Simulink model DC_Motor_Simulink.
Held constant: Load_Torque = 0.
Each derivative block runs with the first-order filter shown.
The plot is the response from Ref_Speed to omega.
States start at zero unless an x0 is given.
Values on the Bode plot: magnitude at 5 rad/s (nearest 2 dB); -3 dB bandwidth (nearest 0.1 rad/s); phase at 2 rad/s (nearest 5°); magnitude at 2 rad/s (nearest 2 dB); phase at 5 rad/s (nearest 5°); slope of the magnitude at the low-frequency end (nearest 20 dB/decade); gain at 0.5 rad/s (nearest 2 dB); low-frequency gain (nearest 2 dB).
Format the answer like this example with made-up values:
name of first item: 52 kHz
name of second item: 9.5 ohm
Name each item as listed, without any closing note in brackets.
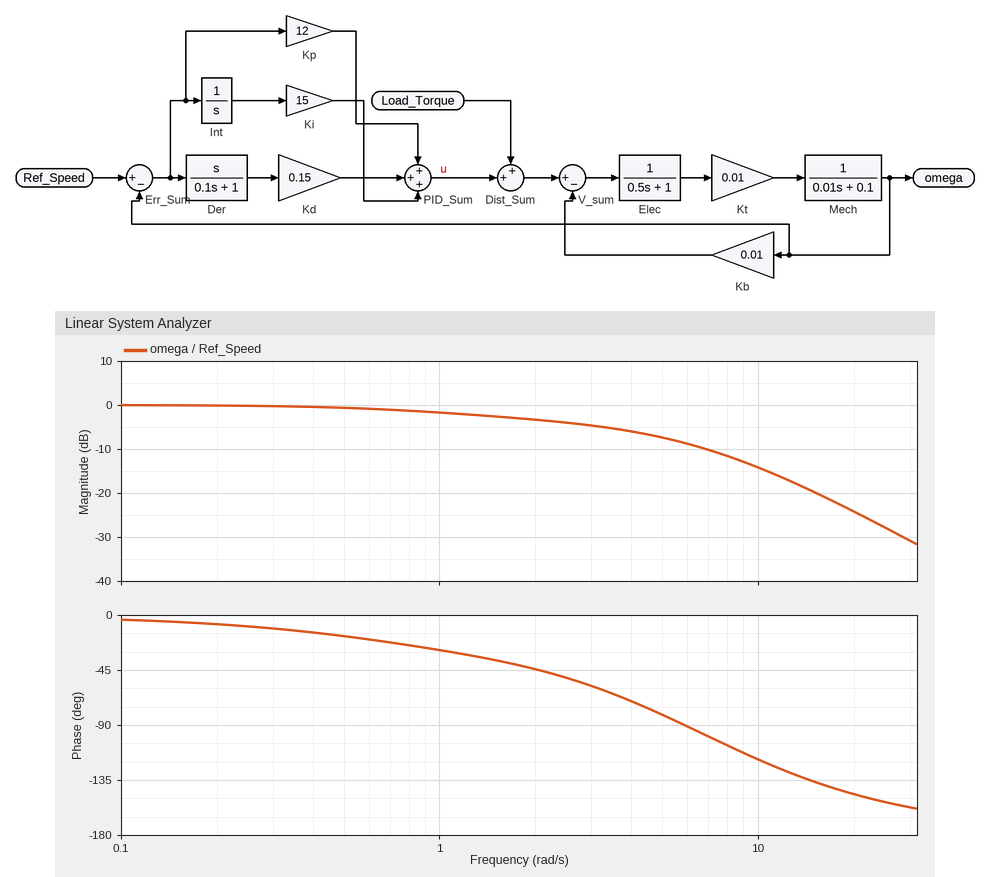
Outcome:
magnitude at 5 rad/s: -8 dB
-3 dB bandwidth: 1.8 rad/s
phase at 2 rad/s: -45°
magnitude at 2 rad/s: -4 dB
phase at 5 rad/s: -80°
slope of the magnitude at the low-frequency end: 0 dB/decade
gain at 0.5 rad/s: 0 dB
low-frequency gain: 0 dB
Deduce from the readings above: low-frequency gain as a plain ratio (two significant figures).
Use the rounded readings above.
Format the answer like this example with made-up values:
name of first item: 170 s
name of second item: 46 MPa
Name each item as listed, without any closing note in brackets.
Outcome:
low-frequency gain as a plain ratio: 1.0
